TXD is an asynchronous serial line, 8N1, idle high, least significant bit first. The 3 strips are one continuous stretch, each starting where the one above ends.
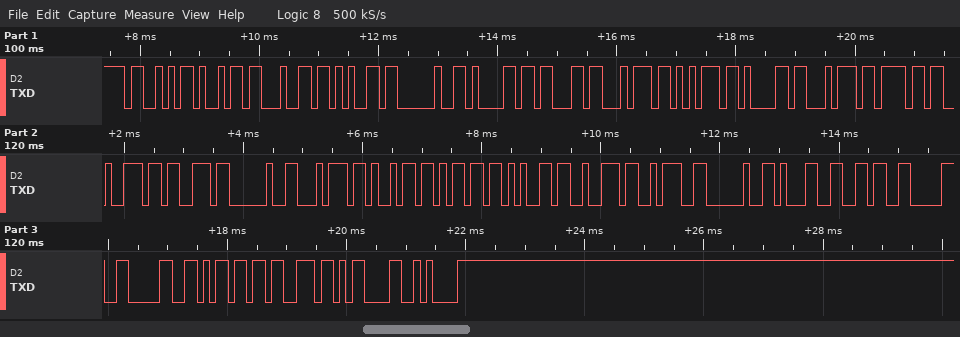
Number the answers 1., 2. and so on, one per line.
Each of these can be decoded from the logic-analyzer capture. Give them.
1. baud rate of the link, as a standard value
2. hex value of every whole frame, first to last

1. 9600 baud
2. 0x53 0x69 0x64 0x65 0x20 0x61 0x63 0x74 0x75 0x61 0x74 0x6F 0x72 0x73 0x20 0x74 0x69 0x6D 0x65 0x72 0x3A 0x20 0x31 0x36 0x30 0x30 0x6D 0x73 0x0D 0x0A
